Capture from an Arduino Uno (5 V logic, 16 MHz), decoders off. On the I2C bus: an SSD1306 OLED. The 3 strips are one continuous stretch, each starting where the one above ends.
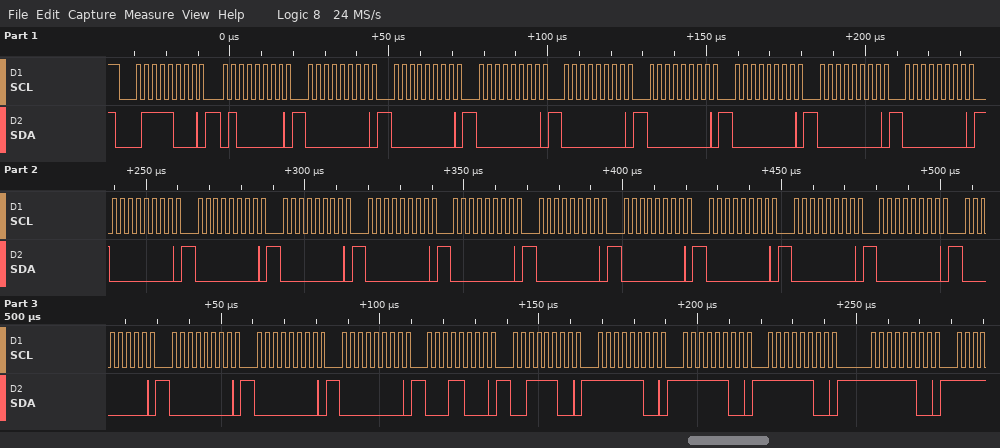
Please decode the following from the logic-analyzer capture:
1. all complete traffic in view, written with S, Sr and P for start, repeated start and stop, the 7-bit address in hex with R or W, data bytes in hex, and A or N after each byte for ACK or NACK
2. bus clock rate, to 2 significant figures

S 3CW A 40 A 00 A 00 A 00 A 00 A 00 A 00 A 00 A 00 A 00 A 00 A 00 A 00 A 00 A 00 A 00 A 00 A 00 A 00 A 00 A 00 A 00 A 00 A 18 A 3C A FC A FC A FC A FC A
400 kHz
